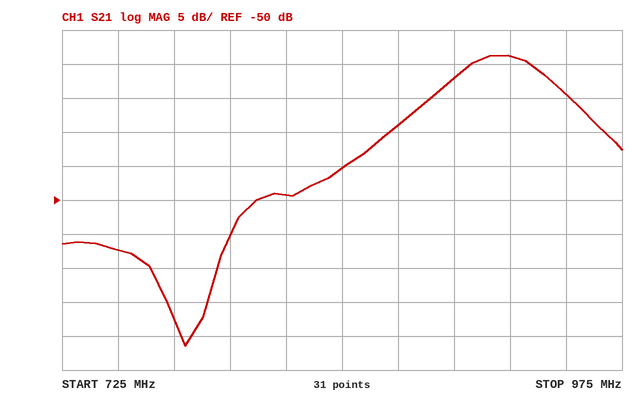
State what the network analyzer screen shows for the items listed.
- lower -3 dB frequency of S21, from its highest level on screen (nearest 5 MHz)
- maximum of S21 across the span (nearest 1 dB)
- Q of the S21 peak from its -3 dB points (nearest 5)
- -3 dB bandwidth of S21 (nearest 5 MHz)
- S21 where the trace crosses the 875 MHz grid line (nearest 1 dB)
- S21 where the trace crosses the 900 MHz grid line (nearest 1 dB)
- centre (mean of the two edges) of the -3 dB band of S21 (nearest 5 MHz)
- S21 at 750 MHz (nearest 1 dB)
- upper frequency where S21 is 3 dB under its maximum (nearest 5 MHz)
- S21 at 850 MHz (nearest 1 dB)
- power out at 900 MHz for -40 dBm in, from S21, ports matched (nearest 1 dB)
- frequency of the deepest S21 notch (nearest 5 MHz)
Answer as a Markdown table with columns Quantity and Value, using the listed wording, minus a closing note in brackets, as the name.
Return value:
| Quantity | Value |
|---|---|
| lower -3 dB frequency of S21, from its highest level on screen | 900 MHz |
| maximum of S21 across the span | -29 dB |
| Q of the S21 peak from its -3 dB points | 25 |
| -3 dB bandwidth of S21 | 40 MHz |
| S21 where the trace crosses the 875 MHz grid line | -39 dB |
| S21 where the trace crosses the 900 MHz grid line | -32 dB |
| centre (mean of the two edges) of the -3 dB band of S21 | 920 MHz |
| S21 at 750 MHz | -57 dB |
| upper frequency where S21 is 3 dB under its maximum | 940 MHz |
| S21 at 850 MHz | -45 dB |
| power out at 900 MHz for -40 dBm in, from S21, ports matched | -72 dBm |
| frequency of the deepest S21 notch | 780 MHz |
